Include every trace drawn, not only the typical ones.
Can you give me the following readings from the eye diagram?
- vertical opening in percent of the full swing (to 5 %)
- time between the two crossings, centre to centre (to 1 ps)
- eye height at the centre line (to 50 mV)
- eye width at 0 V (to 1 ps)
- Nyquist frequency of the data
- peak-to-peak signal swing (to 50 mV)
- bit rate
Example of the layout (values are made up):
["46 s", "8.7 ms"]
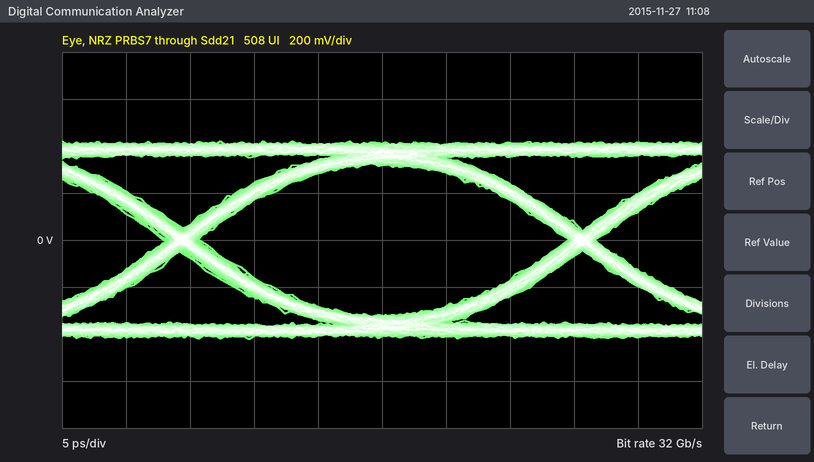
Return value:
["75 %", "31 ps", "650 mV", "29 ps", "16 GHz", "850 mV", "32 Gb/s"]
